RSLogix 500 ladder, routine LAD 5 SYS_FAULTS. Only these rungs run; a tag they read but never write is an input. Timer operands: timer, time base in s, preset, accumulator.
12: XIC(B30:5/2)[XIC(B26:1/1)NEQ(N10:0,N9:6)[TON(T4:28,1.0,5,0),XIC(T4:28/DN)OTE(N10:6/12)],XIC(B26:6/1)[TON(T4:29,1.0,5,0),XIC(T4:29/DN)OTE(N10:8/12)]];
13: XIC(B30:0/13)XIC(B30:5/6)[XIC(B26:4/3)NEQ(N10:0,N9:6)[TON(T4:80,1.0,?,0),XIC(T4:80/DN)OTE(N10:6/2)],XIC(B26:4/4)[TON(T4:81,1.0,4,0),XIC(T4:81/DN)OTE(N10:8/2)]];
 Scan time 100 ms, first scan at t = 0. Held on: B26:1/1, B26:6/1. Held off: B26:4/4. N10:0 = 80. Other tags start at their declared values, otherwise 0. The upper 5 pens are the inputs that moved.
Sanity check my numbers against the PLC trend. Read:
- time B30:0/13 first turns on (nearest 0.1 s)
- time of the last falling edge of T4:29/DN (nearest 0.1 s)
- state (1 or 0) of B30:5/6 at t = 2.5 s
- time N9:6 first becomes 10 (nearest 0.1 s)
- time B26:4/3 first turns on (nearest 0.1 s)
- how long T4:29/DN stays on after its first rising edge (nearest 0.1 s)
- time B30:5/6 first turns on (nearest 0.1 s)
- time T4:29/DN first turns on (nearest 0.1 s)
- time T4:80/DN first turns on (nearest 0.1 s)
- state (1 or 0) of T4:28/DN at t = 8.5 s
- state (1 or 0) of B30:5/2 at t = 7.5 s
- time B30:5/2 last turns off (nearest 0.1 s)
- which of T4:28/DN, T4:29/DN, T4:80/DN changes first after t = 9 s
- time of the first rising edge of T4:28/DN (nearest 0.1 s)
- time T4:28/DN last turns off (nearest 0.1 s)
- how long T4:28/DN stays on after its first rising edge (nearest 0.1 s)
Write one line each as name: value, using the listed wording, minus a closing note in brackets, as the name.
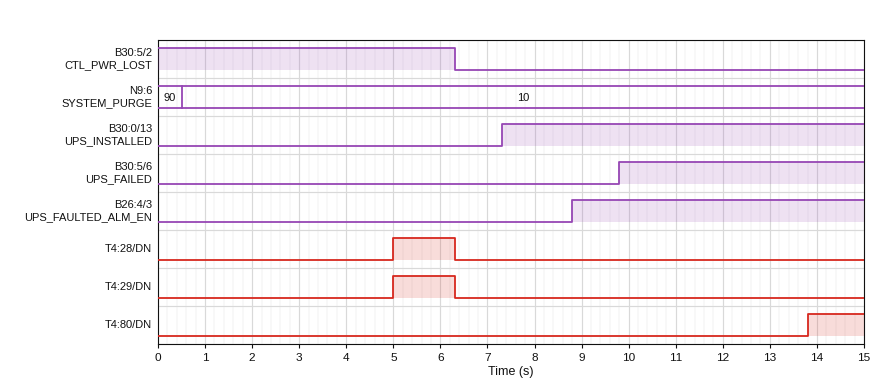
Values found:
time B30:0/13 first turns on: 7.3 s
time of the last falling edge of T4:29/DN: 6.3 s
state (1 or 0) of B30:5/6 at t = 2.5 s: 0
time N9:6 first becomes 10: 0.5 s
time B26:4/3 first turns on: 8.8 s
how long T4:29/DN stays on after its first rising edge: 1.3 s
time B30:5/6 first turns on: 9.8 s
time T4:29/DN first turns on: 5.0 s
time T4:80/DN first turns on: 13.8 s
state (1 or 0) of T4:28/DN at t = 8.5 s: 0
state (1 or 0) of B30:5/2 at t = 7.5 s: 0
time B30:5/2 last turns off: 6.3 s
which of T4:28/DN, T4:29/DN, T4:80/DN changes first after t = 9 s: T4:80/DN
time of the first rising edge of T4:28/DN: 5.0 s
time T4:28/DN last turns off: 6.3 s
how long T4:28/DN stays on after its first rising edge: 1.3 s
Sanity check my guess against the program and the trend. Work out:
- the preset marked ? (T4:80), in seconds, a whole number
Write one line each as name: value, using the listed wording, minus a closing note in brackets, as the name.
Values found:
the preset marked ? (T4:80), in seconds, a whole number: 4 s
